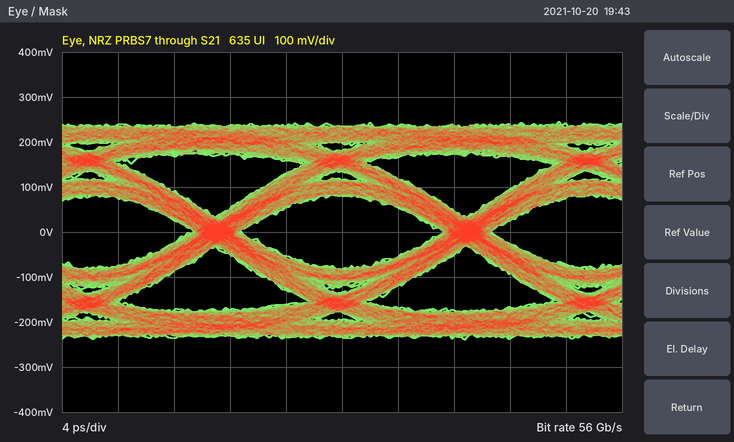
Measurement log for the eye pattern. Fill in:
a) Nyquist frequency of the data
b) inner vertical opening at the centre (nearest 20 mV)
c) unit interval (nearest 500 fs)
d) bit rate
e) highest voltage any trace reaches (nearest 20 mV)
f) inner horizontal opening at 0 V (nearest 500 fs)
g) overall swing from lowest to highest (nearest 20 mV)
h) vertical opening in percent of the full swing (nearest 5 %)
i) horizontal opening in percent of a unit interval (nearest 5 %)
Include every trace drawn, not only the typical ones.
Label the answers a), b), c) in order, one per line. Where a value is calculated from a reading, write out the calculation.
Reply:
a) 28 GHz
b) 160 mV
c) 18.0 ps
d) 56 Gb/s
e) 240 mV
f) 14.5 ps
g) 480 mV
h) 160 mV / 480 mV ≈ 33.3 %, so 35 % to the nearest 5 %
i) 14.5 ps / 18.0 ps ≈ 80.6 %, so 80 % to the nearest 5 %
